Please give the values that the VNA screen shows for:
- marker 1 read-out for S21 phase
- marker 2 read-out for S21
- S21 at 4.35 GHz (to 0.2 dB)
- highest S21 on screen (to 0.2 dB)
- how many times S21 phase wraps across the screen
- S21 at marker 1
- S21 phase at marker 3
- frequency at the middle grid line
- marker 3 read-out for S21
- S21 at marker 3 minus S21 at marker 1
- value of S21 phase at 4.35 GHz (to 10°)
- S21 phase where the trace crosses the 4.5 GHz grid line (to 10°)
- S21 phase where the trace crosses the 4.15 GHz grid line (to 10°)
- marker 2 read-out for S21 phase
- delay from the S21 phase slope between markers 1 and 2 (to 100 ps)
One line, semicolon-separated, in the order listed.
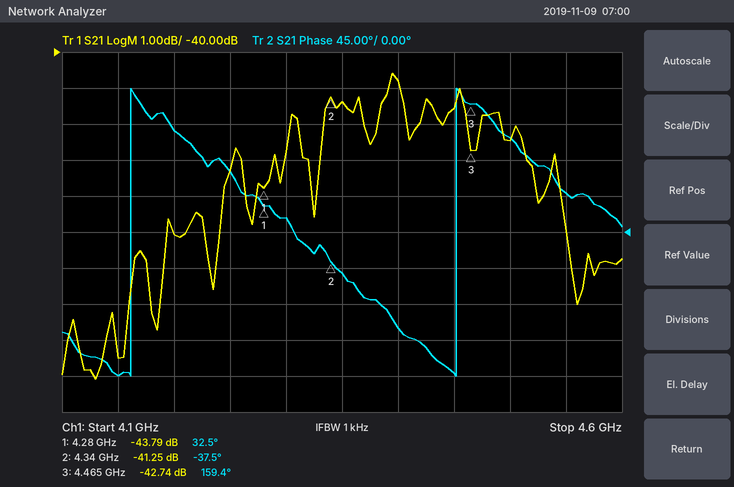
32.5°; -41.25 dB; -41.4 dB; -40.6 dB; 2; -43.79 dB; 159.4°; 4.35 GHz; -42.74 dB; 1.05 dB; -50°; 120°; -180°; -37.5°; 3.2 ns
